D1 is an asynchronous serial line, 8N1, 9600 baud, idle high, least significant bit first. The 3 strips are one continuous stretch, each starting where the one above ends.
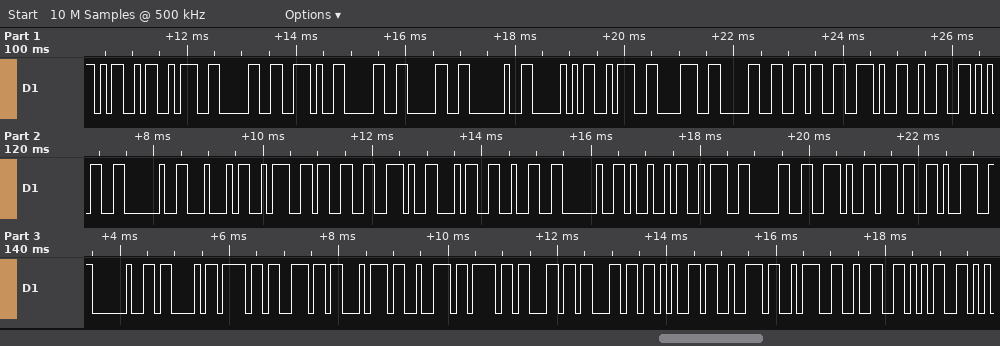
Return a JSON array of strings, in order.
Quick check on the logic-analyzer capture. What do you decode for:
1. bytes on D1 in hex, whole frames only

["0x4D 0x3A 0x30 0x2E 0x30 0x30 0x20 0x50 0x3A 0x38 0x30 0x36 0x2E 0x32 0x35 0x20 0x44 0x3A 0x33 0x2E 0x34 0x32 0x20 0x49 0x3A 0x30 0x2E 0x37 0x39 0x20 0x43 0x6F 0x6E 0x74 0x72 0x6F 0x6C 0x6C 0x65 0x72 0x3A 0x32 0x35"]
